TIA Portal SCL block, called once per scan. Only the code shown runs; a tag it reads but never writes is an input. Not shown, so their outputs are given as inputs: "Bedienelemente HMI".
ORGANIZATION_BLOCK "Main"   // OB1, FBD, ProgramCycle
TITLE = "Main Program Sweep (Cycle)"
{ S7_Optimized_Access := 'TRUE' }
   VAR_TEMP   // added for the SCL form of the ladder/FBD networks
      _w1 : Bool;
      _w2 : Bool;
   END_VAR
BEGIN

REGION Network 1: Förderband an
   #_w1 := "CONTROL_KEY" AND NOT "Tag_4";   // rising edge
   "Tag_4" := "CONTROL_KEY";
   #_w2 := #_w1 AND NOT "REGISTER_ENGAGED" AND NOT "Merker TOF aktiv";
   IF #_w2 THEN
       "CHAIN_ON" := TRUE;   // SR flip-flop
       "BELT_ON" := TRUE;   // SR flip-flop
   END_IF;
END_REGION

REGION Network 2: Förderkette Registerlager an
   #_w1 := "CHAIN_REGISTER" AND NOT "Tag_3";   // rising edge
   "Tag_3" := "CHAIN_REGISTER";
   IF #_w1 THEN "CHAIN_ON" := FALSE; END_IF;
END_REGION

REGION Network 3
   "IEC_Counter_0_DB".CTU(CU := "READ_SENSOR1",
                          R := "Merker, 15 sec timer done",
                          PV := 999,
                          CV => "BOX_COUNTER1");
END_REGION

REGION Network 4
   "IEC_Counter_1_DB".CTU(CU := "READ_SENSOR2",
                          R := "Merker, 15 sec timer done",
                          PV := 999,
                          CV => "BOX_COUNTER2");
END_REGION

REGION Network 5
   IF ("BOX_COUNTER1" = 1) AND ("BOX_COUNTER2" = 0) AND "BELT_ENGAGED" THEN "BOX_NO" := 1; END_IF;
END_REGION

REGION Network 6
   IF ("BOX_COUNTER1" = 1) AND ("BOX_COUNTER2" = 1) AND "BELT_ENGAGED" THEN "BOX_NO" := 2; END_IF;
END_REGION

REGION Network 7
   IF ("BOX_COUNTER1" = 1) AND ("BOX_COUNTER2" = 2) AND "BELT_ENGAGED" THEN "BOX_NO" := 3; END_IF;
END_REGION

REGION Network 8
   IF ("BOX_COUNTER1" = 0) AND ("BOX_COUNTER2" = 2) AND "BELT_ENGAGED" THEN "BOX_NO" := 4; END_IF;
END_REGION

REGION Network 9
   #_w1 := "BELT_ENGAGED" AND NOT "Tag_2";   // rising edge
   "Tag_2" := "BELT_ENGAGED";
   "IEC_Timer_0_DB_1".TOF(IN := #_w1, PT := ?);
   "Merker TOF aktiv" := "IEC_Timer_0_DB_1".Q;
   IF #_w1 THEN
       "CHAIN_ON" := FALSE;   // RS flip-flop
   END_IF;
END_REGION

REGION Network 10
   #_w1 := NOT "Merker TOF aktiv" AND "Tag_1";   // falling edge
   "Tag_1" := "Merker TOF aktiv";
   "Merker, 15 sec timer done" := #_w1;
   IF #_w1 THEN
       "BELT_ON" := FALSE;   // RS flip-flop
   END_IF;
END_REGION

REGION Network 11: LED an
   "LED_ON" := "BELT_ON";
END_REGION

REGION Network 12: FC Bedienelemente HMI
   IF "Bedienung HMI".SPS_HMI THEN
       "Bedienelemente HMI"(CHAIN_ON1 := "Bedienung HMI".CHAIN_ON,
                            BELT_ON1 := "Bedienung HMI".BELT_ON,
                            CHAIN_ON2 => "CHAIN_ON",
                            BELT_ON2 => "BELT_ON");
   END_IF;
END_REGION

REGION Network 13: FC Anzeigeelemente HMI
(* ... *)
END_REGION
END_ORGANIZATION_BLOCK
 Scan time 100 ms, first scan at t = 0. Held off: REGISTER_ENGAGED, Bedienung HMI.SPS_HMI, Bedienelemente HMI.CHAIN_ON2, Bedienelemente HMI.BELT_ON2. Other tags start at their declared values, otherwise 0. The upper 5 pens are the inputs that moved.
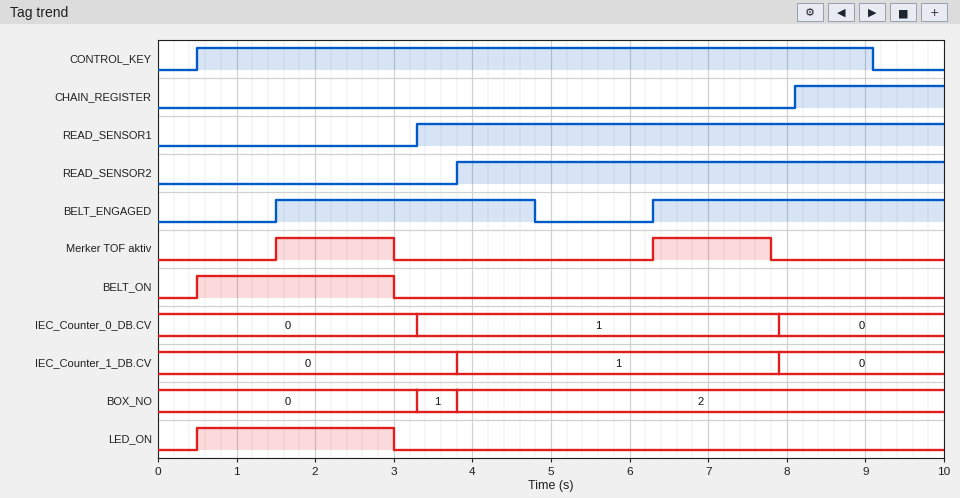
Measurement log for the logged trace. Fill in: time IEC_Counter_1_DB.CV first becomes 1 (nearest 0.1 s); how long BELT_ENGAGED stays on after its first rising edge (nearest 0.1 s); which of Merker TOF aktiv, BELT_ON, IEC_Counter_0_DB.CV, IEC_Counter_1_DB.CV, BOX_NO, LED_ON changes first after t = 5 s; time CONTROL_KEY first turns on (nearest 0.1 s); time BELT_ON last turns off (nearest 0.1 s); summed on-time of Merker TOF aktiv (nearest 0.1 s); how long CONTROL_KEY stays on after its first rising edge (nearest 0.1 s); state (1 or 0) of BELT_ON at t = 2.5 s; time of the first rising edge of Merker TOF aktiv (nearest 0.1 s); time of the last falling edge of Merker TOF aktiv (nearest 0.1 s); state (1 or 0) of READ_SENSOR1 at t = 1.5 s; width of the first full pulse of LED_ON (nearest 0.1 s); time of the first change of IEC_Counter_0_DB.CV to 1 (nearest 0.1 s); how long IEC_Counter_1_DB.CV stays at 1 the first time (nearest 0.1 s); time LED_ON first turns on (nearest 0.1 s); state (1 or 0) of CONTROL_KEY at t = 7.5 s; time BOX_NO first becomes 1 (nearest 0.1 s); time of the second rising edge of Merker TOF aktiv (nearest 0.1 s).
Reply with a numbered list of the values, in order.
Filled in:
1. 3.8 s
2. 3.3 s
3. Merker TOF aktiv
4. 0.5 s
5. 3.0 s
6. 3.0 s
7. 8.6 s
8. 1
9. 1.5 s
10. 7.8 s
11. 0
12. 2.5 s
13. 3.3 s
14. 4.1 s
15. 0.5 s
16. 1
17. 3.3 s
18. 6.3 s
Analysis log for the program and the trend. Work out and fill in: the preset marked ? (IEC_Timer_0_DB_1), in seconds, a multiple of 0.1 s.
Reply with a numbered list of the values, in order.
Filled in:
1. 1.4 s
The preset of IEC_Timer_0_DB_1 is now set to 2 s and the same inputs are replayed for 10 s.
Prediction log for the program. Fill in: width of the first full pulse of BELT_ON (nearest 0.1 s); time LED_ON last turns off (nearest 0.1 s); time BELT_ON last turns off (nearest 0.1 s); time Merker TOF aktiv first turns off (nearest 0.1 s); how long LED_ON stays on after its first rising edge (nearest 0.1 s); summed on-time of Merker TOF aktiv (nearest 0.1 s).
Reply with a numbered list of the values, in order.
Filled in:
1. 3.1 s
2. 3.6 s
3. 3.6 s
4. 3.6 s
5. 3.1 s
6. 4.2 s
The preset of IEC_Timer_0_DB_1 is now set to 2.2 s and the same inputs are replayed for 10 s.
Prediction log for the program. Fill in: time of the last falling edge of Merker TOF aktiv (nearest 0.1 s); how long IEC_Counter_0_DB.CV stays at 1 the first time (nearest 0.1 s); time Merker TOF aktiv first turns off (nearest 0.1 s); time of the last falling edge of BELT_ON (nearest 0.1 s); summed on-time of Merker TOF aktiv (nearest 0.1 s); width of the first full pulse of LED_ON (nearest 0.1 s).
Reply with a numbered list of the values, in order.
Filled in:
1. 8.6 s
2. 0.6 s
3. 3.8 s
4. 3.8 s
5. 4.6 s
6. 3.3 s
